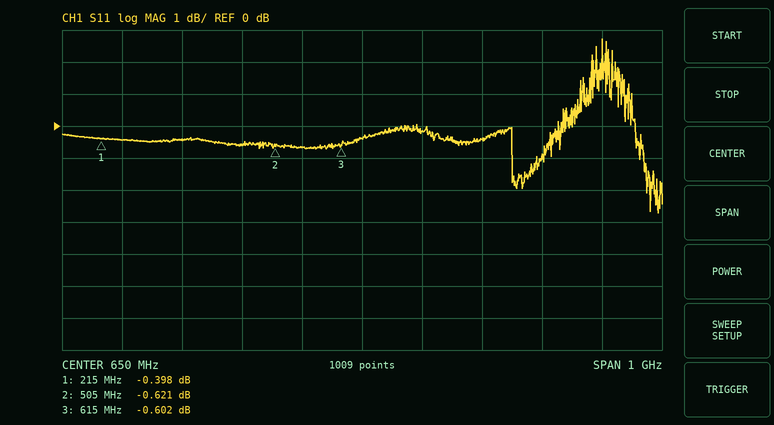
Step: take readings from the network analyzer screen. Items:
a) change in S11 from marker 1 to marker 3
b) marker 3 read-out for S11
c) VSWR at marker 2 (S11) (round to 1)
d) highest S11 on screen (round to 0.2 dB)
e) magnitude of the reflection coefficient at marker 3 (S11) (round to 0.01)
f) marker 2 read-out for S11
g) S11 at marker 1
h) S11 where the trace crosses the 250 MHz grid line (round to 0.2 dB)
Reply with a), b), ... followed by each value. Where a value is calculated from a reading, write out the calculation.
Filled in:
a) -0.602 − (-0.398) = -0.204 dB
b) -0.602 dB
c) (1 + 0.9310)/(1 − 0.9310) ≈ 28
d) 2.8 dB
e) 10^(-0.602/20) ≈ 0.93
f) -0.621 dB
g) -0.398 dB
h) -0.4 dB
